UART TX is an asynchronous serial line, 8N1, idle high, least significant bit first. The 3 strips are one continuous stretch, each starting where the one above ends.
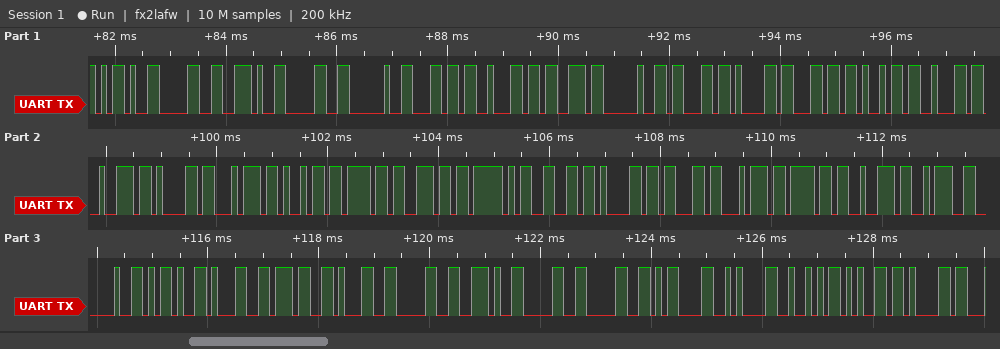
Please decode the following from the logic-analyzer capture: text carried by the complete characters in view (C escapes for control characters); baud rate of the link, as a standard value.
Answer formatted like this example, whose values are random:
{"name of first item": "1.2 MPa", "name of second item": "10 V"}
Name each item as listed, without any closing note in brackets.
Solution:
{"text carried by the complete characters in view": "\"-0.0 lbs calibration_factor: -1710.00\\r\\nRea\"", "baud rate of the link, as a standard value": "9600 baud"}
